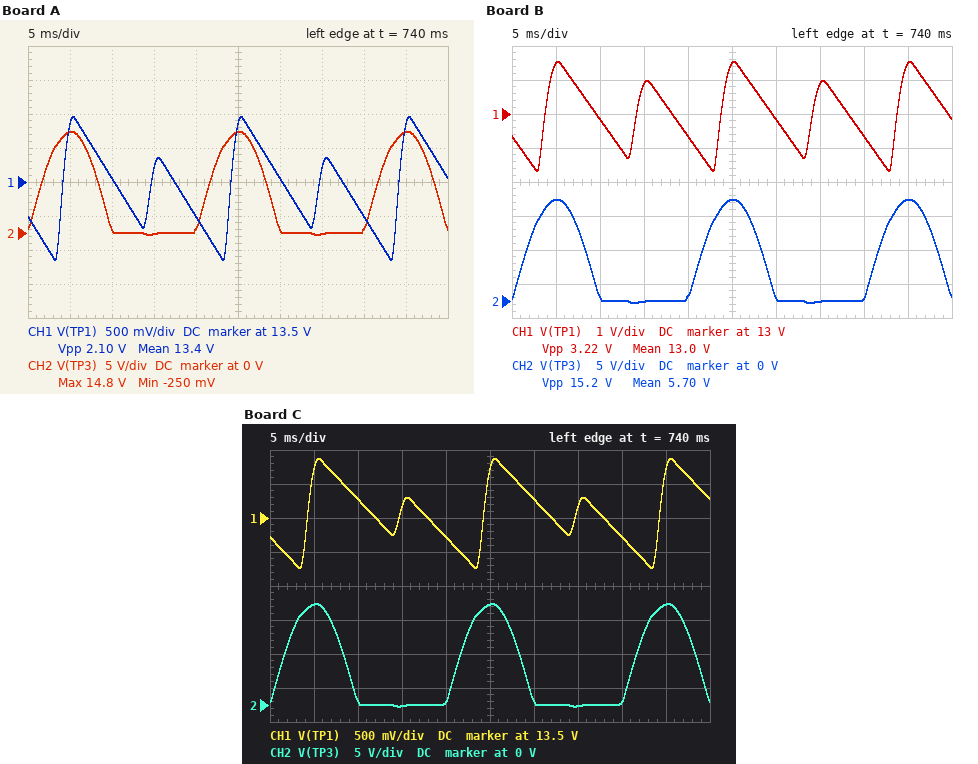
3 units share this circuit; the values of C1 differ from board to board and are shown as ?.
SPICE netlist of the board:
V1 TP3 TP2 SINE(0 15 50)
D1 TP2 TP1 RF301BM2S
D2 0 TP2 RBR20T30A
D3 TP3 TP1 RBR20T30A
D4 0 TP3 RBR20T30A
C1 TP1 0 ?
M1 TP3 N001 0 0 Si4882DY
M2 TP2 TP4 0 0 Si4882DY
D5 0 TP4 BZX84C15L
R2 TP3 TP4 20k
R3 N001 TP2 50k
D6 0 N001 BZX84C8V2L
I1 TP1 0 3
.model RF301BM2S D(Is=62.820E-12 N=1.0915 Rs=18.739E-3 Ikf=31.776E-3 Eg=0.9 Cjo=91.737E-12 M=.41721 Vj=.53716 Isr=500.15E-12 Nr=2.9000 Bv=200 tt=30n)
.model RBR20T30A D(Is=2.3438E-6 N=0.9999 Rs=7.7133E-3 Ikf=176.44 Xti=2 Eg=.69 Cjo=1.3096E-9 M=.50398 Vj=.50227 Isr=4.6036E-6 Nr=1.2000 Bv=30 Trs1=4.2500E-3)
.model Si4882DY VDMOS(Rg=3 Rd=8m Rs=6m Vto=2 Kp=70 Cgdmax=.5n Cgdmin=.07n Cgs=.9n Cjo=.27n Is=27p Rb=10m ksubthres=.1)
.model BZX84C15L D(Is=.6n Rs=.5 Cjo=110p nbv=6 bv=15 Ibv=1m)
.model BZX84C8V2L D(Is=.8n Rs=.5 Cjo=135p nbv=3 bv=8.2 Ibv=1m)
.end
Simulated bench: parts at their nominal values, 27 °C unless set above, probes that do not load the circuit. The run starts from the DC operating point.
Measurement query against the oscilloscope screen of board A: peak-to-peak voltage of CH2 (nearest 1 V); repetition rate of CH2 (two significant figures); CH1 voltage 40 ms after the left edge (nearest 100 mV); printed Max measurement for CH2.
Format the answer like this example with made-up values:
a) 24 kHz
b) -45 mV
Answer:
a) 15 V
b) 50 Hz
c) 13.0 V
d) 14.8 V
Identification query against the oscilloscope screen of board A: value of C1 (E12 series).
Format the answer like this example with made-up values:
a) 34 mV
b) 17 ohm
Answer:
a) 15 mF
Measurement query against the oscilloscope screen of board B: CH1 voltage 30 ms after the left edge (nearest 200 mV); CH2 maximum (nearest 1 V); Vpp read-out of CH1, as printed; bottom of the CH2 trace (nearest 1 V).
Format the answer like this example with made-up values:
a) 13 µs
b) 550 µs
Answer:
a) 12.8 V
b) 15 V
c) 3.22 V
d) 0 V
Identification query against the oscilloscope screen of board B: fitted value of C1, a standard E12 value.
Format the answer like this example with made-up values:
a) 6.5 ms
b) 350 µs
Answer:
a) 8.2 mF
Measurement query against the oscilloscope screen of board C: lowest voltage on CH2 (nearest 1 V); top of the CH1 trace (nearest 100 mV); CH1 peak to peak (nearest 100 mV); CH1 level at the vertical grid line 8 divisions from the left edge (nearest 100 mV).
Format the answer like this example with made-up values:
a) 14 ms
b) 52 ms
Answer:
a) 0 V
b) 14.4 V
c) 1.6 V
d) 13.2 V
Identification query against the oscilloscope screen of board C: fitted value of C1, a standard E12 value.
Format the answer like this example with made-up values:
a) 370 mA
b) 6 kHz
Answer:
a) 22 mF
